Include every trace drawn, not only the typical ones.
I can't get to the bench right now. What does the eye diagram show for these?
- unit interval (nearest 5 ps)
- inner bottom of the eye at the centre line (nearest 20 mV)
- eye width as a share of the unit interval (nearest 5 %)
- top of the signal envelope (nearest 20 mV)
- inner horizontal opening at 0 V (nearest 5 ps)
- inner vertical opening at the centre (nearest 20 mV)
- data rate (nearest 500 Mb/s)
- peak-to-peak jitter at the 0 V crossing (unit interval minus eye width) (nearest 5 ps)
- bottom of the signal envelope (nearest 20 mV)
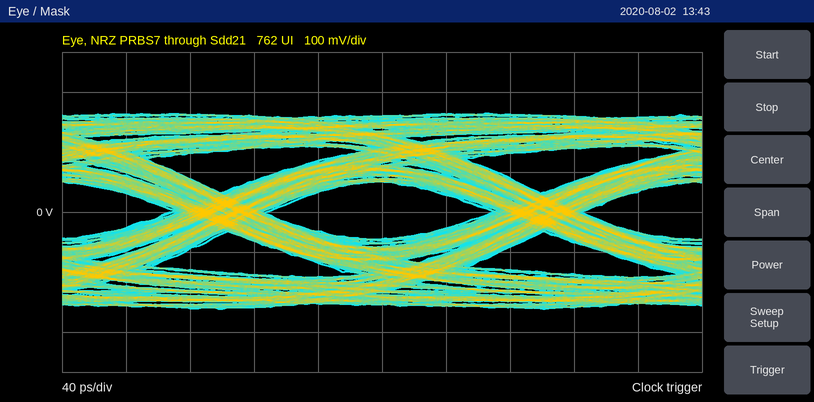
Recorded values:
200 ps
-60 mV
70 %
240 mV
140 ps
140 mV
5.0 Gb/s
60 ps
-240 mV
